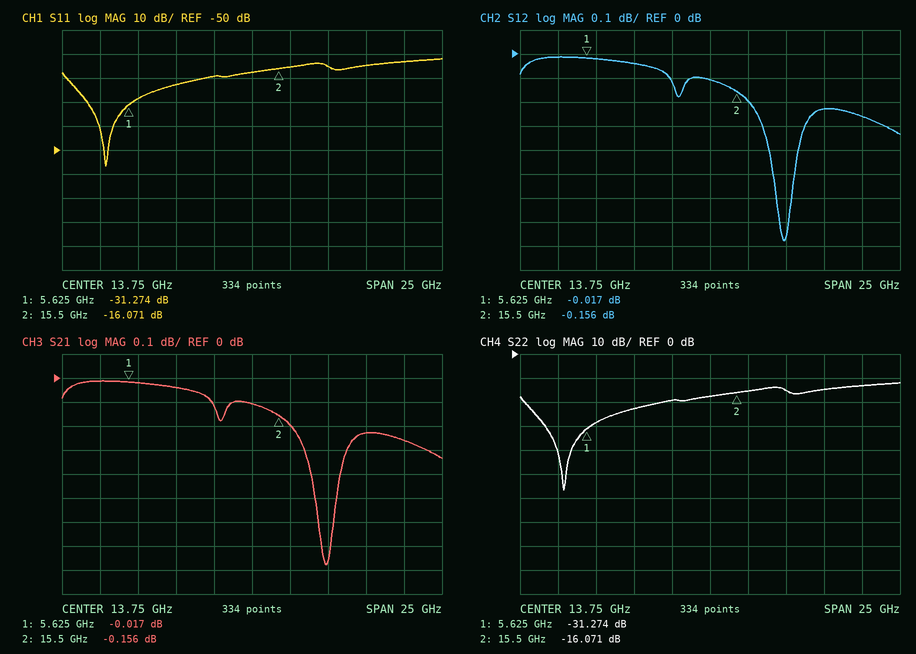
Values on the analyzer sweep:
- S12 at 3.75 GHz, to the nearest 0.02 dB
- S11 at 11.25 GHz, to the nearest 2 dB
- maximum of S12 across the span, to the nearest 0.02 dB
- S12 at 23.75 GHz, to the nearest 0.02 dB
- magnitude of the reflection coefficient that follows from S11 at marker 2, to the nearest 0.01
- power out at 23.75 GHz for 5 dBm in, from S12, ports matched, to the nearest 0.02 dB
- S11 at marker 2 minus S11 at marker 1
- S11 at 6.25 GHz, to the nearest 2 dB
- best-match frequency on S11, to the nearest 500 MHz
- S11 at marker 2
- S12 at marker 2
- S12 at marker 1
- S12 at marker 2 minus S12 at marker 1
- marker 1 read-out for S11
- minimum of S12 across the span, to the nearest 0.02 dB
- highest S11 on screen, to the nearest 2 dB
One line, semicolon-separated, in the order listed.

-0.02 dB; -20 dB; -0.02 dB; -0.26 dB; 0.16; 4.74 dBm; 15.203 dB; -28 dB; 4.0 GHz; -16.071 dB; -0.156 dB; -0.017 dB; -0.139 dB; -31.274 dB; -0.78 dB; -12 dB
